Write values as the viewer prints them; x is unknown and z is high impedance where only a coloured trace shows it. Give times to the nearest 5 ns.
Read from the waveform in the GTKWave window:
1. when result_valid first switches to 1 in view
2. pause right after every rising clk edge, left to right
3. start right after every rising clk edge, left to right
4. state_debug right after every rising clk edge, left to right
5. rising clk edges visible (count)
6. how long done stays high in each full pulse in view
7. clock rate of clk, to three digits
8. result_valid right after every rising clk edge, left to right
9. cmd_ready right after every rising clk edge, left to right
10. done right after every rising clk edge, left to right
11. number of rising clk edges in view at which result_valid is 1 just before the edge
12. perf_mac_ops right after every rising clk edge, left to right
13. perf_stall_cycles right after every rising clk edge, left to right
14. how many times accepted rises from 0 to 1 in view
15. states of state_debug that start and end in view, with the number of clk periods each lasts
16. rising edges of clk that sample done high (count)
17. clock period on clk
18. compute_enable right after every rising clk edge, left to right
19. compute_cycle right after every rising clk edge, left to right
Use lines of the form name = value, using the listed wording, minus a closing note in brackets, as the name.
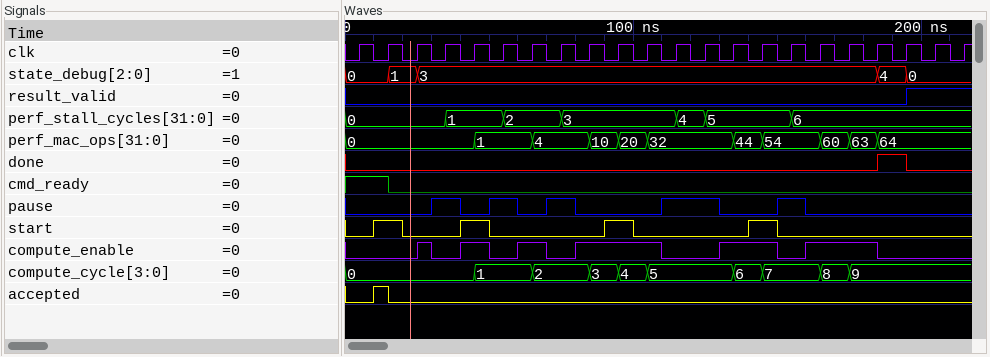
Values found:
when result_valid first switches to 1 in view = 195 ns
pause right after every rising clk edge, left to right = 0 0 0 1 0 1 0 1 0 0 0 1 1 0 0 1 0 0 0 0 0 0
start right after every rising clk edge, left to right = 0 1 0 0 1 0 0 0 0 1 0 0 0 0 1 0 0 0 0 0 0 0
state_debug right after every rising clk edge, left to right = 0, 1, 3, 3, 3, 3, 3, 3, 3, 3, 3, 3, 3, 3, 3, 3, 3, 3, 4, 0, 0, 0
rising clk edges visible = 22
how long done stays high in each full pulse in view = 10 ns
clock rate of clk, to three digits = 100 MHz
result_valid right after every rising clk edge, left to right = 0 0 0 0 0 0 0 0 0 0 0 0 0 0 0 0 0 0 0 1 1 1
cmd_ready right after every rising clk edge, left to right = 1 0 0 0 0 0 0 0 0 0 0 0 0 0 0 0 0 0 0 0 0 0
done right after every rising clk edge, left to right = 0 0 0 0 0 0 0 0 0 0 0 0 0 0 0 0 0 0 1 0 0 0
number of rising clk edges in view at which result_valid is 1 just before the edge = 2
perf_mac_ops right after every rising clk edge, left to right = 0, 0, 0, 0, 1, 1, 4, 4, 10, 20, 32, 32, 32, 44, 54, 54, 60, 63, 64, 64, 64, 64
perf_stall_cycles right after every rising clk edge, left to right = 0, 0, 0, 1, 1, 2, 2, 3, 3, 3, 3, 4, 5, 5, 5, 6, 6, 6, 6, 6, 6, 6
how many times accepted rises from 0 to 1 in view = 1
states of state_debug that start and end in view, with the number of clk periods each lasts = 1: 1, 3: 16, 4: 1
rising edges of clk that sample done high = 1
clock period on clk = 10 ns
compute_enable right after every rising clk edge, left to right = 0 0 1 0 1 0 1 0 1 1 1 0 0 1 1 0 1 1 0 0 0 0
compute_cycle right after every rising clk edge, left to right = 0, 0, 0, 0, 1, 1, 2, 2, 3, 4, 5, 5, 5, 6, 7, 7, 8, 9, 9, 9, 9, 9
